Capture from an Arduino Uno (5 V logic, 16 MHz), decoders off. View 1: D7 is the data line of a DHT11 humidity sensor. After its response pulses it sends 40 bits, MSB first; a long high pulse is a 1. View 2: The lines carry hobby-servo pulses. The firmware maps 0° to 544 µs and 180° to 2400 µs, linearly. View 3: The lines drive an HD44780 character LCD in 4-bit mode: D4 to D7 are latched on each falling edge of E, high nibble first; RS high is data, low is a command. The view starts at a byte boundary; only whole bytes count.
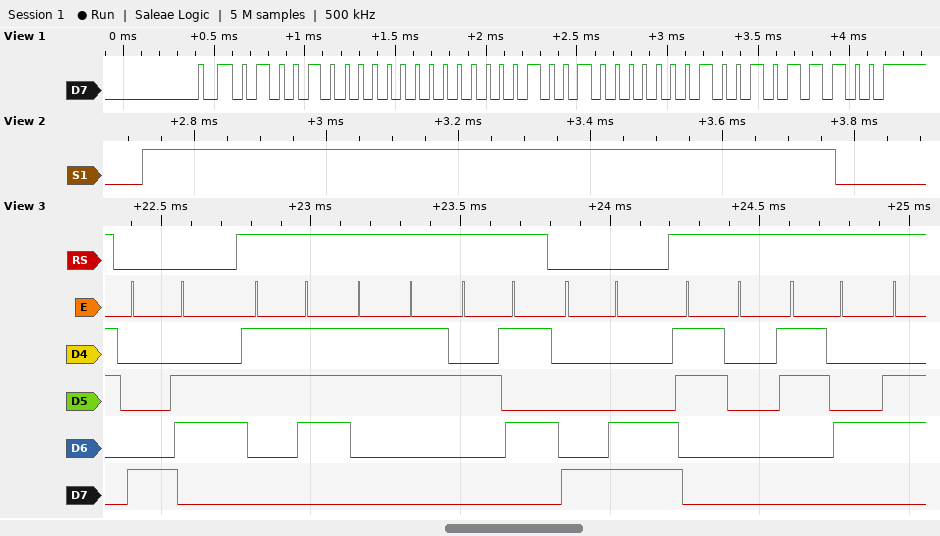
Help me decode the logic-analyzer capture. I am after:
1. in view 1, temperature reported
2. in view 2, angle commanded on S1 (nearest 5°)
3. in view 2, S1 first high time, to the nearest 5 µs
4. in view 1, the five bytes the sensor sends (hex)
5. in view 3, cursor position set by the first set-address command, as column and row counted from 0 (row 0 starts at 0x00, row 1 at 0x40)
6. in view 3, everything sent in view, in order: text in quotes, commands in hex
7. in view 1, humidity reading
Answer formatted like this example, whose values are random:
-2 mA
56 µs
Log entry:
18.2 °C
50°
1050 µs
48 00 12 02 5C
column 6, row 0
0x86 "73%" 0x8C "04"
72 %
